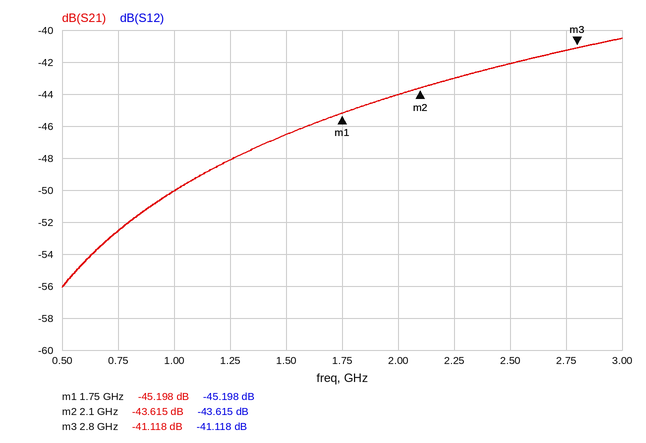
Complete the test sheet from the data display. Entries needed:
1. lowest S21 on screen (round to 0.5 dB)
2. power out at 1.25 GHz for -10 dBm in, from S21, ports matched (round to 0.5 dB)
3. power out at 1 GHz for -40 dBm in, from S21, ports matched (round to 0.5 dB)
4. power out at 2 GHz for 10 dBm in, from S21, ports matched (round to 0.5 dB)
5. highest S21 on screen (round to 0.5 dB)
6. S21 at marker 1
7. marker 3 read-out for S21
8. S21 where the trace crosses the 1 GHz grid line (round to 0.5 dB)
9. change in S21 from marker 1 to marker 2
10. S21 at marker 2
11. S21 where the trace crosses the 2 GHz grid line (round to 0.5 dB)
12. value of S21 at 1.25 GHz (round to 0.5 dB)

-56.0 dB
-58.0 dBm
-90.0 dBm
-34.0 dBm
-40.5 dB
-45.198 dB
-41.118 dB
-50.0 dB
1.583 dB
-43.615 dB
-44.0 dB
-48.0 dB
